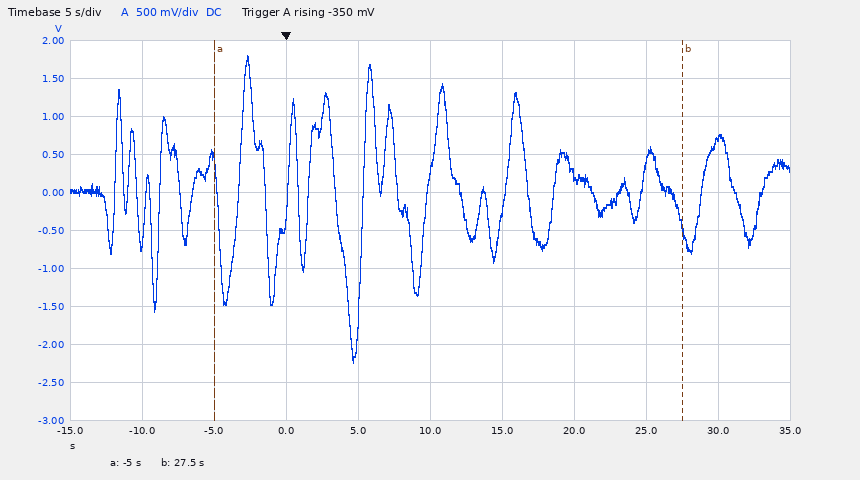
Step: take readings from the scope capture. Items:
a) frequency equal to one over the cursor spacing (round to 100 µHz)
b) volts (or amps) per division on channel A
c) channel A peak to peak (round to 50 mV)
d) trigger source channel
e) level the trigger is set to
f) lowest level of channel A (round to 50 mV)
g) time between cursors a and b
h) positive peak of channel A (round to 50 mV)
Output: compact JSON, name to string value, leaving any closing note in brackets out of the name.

{"frequency equal to one over the cursor spacing": "30.8 mHz", "volts (or amps) per division on channel A": "500 mV", "channel A peak to peak": "4.05 V", "trigger source channel": "channel A", "level the trigger is set to": "-350 mV", "lowest level of channel A": "-2.25 V", "time between cursors a and b": "32.5 s", "positive peak of channel A": "1.80 V"}
